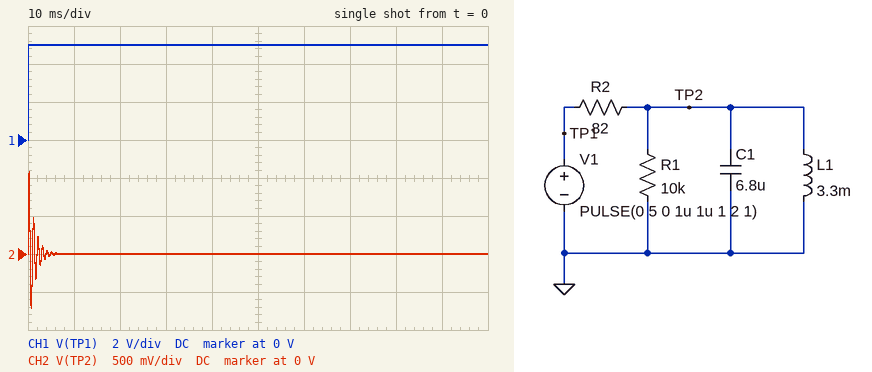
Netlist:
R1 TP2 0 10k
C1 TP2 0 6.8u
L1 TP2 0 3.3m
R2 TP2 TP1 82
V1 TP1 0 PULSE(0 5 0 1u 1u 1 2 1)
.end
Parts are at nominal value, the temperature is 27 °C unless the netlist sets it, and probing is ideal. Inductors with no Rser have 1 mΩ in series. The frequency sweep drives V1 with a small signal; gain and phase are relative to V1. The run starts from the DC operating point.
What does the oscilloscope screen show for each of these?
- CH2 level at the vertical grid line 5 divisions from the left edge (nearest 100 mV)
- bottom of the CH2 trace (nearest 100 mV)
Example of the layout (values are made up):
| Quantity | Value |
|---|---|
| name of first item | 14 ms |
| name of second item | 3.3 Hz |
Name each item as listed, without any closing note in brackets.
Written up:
| Quantity | Value |
|---|---|
| CH2 level at the vertical grid line 5 divisions from the left edge | 0 V |
| bottom of the CH2 trace | -700 mV |
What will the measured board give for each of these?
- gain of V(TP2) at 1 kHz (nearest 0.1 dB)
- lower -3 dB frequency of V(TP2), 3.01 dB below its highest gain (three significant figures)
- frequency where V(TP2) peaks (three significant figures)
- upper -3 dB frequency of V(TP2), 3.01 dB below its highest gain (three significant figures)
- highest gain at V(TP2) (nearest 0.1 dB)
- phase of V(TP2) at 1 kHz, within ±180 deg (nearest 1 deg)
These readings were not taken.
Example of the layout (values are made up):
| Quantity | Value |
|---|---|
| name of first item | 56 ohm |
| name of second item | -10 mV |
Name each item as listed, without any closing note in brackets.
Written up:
| Quantity | Value |
|---|---|
| gain of V(TP2) at 1 kHz | -0.9 dB |
| lower -3 dB frequency of V(TP2), 3.01 dB below its highest gain | 928 Hz |
| frequency where V(TP2) peaks | 1.06 kHz |
| upper -3 dB frequency of V(TP2), 3.01 dB below its highest gain | 1.22 kHz |
| highest gain at V(TP2) | -0.1 dB |
| phase of V(TP2) at 1 kHz, within ±180 deg | 24 deg |
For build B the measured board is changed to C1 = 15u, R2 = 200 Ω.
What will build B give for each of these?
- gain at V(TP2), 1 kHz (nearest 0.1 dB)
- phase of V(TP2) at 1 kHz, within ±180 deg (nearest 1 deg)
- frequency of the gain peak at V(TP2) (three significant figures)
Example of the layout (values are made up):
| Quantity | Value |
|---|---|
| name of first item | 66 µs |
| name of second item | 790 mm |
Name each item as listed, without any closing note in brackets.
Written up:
| Quantity | Value |
|---|---|
| gain at V(TP2), 1 kHz | -19.3 dB |
| phase of V(TP2) at 1 kHz, within ±180 deg | -84 deg |
| frequency of the gain peak at V(TP2) | 715 Hz |
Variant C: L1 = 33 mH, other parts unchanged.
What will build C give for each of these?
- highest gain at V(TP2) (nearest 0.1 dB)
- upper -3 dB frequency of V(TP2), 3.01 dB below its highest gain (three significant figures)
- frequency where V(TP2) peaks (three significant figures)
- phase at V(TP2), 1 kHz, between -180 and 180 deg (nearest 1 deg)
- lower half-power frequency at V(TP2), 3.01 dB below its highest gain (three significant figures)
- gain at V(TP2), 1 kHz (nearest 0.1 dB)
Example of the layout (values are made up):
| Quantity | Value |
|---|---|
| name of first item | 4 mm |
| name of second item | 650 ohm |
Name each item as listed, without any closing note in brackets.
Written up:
| Quantity | Value |
|---|---|
| highest gain at V(TP2) | -0.1 dB |
| upper -3 dB frequency of V(TP2), 3.01 dB below its highest gain | 509 Hz |
| frequency where V(TP2) peaks | 336 Hz |
| phase at V(TP2), 1 kHz, between -180 and 180 deg | -72 deg |
| lower half-power frequency at V(TP2), 3.01 dB below its highest gain | 222 Hz |
| gain at V(TP2), 1 kHz | -10.3 dB |
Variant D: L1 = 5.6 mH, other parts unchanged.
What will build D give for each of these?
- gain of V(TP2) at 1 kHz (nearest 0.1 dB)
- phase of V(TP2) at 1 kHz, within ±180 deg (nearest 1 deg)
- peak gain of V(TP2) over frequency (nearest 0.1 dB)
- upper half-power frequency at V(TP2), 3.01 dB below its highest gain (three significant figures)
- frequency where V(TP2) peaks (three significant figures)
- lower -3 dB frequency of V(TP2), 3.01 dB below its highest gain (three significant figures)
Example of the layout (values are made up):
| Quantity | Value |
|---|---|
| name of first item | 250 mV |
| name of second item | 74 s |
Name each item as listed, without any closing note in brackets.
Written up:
| Quantity | Value |
|---|---|
| gain of V(TP2) at 1 kHz | -3.8 dB |
| phase of V(TP2) at 1 kHz, within ±180 deg | -49 deg |
| peak gain of V(TP2) over frequency | -0.1 dB |
| upper half-power frequency at V(TP2), 3.01 dB below its highest gain | 972 Hz |
| frequency where V(TP2) peaks | 816 Hz |
| lower -3 dB frequency of V(TP2), 3.01 dB below its highest gain | 684 Hz |
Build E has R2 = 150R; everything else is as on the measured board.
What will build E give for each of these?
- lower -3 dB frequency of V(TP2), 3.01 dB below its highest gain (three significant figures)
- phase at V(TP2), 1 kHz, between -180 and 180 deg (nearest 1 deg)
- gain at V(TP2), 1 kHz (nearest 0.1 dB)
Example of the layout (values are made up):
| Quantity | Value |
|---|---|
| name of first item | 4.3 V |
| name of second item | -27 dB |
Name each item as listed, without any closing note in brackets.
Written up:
| Quantity | Value |
|---|---|
| lower -3 dB frequency of V(TP2), 3.01 dB below its highest gain | 986 Hz |
| phase at V(TP2), 1 kHz, between -180 and 180 deg | 39 deg |
| gain at V(TP2), 1 kHz | -2.3 dB |
